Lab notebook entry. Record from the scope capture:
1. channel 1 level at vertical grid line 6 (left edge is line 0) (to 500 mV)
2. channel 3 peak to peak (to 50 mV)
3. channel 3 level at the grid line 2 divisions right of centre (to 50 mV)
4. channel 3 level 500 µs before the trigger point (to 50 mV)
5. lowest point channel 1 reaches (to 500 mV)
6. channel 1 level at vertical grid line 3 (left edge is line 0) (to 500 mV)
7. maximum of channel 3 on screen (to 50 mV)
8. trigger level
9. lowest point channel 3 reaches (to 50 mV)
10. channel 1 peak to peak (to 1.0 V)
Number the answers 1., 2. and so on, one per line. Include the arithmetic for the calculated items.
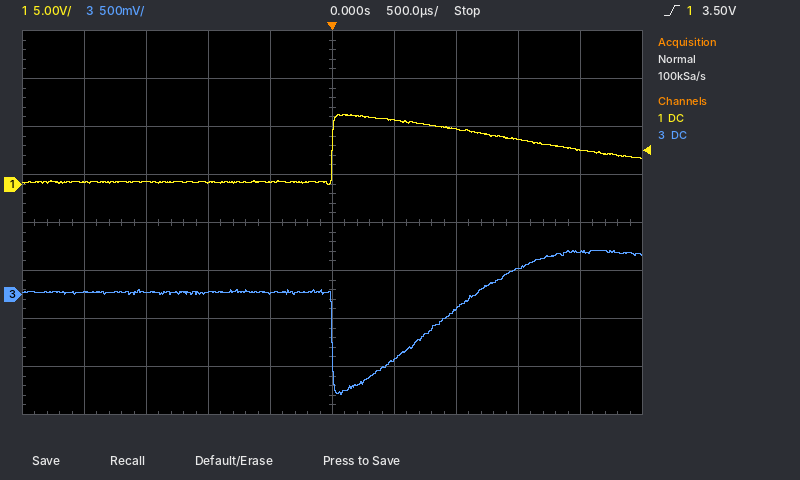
1. 6.5 V
2. 450 mV − (-1.05 V) = 1.50 V
3. -150 mV
4. 0 mV
5. 0.0 V
6. 0.0 V
7. 450 mV
8. 3.50 V
9. -1.05 V
10. 7.0 V
